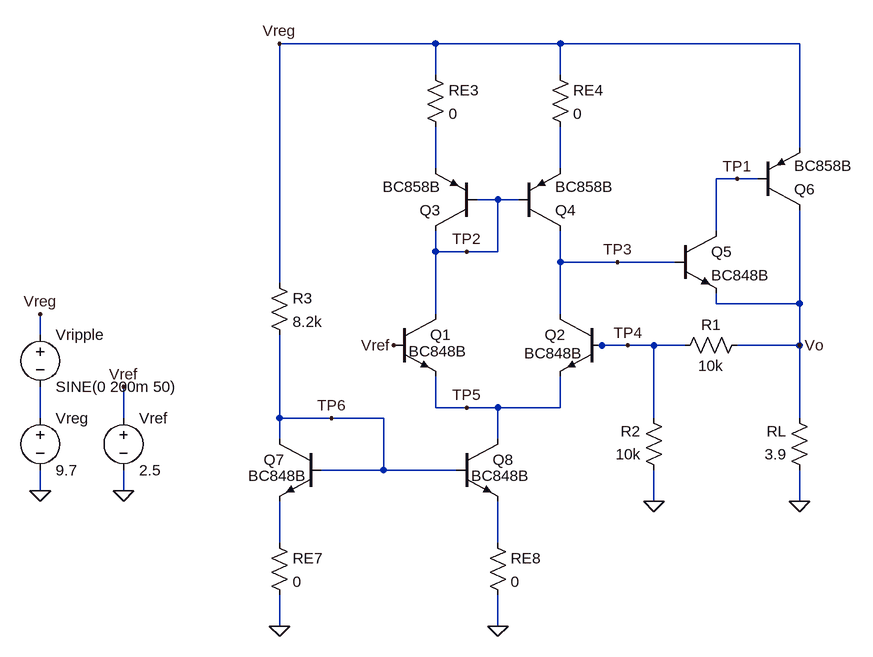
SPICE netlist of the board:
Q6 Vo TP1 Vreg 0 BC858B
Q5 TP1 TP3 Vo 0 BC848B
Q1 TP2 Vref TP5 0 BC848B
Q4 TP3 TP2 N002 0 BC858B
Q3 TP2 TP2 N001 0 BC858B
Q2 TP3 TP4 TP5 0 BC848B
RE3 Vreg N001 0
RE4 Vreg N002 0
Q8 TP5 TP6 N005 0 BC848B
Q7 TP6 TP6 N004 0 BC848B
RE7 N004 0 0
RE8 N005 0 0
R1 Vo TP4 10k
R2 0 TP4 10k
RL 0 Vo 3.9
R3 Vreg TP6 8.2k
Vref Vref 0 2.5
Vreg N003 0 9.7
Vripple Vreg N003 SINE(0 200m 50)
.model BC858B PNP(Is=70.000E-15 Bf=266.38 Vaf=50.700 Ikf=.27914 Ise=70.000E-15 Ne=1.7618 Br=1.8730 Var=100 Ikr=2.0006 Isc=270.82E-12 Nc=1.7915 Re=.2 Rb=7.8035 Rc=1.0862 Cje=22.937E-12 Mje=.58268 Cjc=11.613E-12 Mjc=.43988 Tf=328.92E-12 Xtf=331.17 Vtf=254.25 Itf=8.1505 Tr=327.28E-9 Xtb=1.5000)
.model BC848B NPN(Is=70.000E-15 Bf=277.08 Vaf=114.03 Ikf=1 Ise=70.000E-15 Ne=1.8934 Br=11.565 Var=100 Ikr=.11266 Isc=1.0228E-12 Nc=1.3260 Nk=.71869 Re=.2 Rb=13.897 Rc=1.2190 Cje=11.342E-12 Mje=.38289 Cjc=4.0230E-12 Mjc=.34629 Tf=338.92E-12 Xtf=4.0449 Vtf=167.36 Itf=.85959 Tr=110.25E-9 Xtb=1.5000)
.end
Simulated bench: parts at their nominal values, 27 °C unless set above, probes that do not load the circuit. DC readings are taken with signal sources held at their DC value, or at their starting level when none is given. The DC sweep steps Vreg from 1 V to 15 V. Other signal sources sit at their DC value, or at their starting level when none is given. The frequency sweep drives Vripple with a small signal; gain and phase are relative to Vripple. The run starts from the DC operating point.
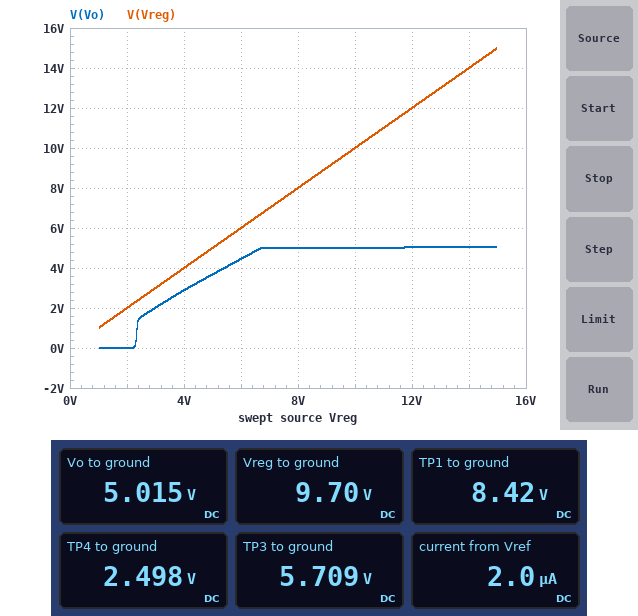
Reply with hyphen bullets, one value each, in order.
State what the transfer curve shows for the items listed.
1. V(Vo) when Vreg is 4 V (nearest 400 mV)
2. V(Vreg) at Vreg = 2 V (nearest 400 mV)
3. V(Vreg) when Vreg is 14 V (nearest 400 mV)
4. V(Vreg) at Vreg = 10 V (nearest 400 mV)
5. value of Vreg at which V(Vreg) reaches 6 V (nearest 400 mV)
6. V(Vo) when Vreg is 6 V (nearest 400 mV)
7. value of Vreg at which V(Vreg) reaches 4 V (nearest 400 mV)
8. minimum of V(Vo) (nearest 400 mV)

- 2.8 V
- 2.0 V
- 14.0 V
- 10.0 V
- 6.0 V
- 4.4 V
- 4.0 V
- 0 V
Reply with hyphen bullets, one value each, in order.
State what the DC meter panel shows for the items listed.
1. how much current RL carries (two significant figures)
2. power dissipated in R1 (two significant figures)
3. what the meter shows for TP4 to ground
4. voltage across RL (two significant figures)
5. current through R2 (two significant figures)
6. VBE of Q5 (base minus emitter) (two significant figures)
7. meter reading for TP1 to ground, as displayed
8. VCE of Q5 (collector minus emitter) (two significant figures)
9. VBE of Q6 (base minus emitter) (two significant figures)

- 1.3 A
- 630 µW
- 2.498 V
- 5.0 V
- 250 µA
- 690 mV
- 8.42 V
- 3.4 V
- -1.3 V
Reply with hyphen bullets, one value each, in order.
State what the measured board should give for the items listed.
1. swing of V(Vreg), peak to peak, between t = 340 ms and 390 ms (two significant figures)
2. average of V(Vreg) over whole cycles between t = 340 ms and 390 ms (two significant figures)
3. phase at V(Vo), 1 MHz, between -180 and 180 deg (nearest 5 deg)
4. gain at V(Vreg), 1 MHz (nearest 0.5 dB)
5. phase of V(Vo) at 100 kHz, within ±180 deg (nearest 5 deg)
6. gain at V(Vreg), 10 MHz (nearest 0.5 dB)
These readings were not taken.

- 400 mV
- 9.7 V
- 85 deg
- 0 dB
- 20 deg
- 0 dB
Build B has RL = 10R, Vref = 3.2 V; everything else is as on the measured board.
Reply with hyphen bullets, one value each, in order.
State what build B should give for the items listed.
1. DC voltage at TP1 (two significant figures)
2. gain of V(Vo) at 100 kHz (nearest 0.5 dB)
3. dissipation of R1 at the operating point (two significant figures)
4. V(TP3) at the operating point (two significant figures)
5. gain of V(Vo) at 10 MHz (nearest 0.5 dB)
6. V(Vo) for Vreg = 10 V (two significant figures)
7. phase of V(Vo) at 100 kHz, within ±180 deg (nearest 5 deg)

- 8.7 V
- -47.0 dB
- 1.0 mW
- 7.1 V
- -6.5 dB
- 6.4 V
- 25 deg
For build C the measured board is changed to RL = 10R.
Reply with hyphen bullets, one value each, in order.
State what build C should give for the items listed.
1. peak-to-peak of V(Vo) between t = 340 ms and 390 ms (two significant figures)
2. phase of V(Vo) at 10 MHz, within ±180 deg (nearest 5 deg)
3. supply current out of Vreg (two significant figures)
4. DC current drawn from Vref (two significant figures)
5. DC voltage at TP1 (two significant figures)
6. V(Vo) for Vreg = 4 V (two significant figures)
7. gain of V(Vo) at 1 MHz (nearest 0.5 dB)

- 1.6 mV
- 60 deg
- 510 mA
- 1.9 µA
- 8.8 V
- 3.1 V
- -35.5 dB
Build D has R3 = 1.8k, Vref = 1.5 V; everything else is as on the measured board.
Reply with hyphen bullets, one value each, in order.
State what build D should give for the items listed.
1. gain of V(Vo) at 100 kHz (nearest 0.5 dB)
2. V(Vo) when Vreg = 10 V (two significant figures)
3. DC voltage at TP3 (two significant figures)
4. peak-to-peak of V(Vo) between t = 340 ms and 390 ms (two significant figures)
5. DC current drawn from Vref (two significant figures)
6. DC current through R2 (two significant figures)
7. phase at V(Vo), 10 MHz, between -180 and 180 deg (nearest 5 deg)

- -38.0 dB
- 3.1 V
- 3.8 V
- 5.0 mV
- 8.2 µA
- 150 µA
- 30 deg
